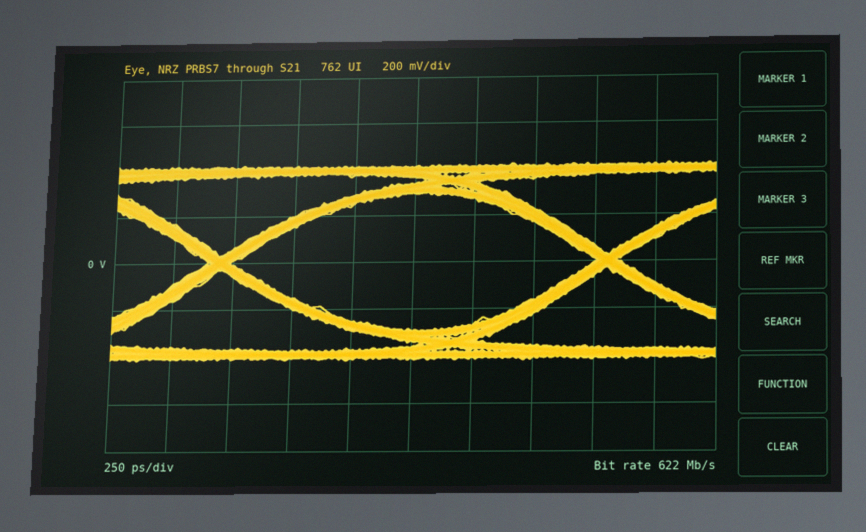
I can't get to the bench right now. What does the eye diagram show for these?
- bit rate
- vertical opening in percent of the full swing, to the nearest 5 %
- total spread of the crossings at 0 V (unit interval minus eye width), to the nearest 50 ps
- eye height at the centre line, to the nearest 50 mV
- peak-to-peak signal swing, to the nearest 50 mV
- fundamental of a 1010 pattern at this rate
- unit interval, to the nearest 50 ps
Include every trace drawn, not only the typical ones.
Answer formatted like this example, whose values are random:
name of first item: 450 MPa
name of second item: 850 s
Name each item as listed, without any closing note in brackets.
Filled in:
bit rate: 622 Mb/s
vertical opening in percent of the full swing, to the nearest 5 %: 70 %
total spread of the crossings at 0 V (unit interval minus eye width), to the nearest 50 ps: 100 ps
eye height at the centre line, to the nearest 50 mV: 600 mV
peak-to-peak signal swing, to the nearest 50 mV: 850 mV
fundamental of a 1010 pattern at this rate: 311 MHz
unit interval, to the nearest 50 ps: 1.60 ns
